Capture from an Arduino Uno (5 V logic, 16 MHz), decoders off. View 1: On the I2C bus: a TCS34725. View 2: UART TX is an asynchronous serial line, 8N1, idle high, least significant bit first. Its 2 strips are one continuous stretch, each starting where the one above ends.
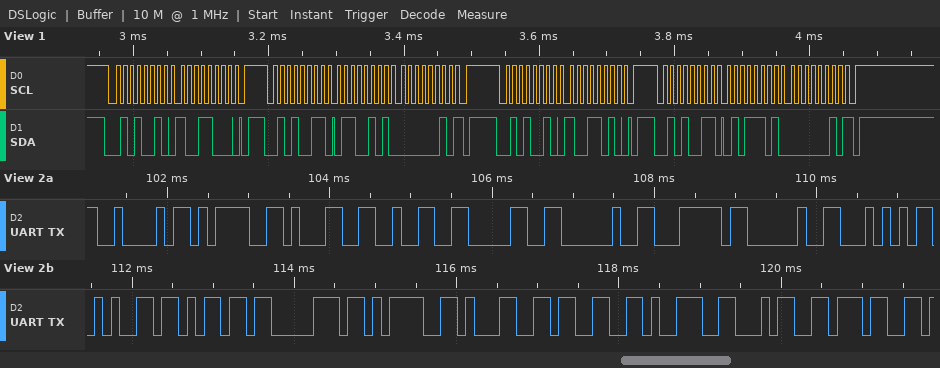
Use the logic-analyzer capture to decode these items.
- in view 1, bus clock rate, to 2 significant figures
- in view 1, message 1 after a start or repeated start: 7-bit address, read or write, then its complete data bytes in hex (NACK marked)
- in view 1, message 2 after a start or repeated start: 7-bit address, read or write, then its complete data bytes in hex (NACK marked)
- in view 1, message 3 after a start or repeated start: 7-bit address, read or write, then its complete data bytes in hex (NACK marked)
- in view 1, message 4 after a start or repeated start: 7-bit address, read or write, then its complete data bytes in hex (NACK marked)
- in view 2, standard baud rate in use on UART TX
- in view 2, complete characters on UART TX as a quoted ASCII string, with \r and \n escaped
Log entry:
100 kHz
0x29 write: 98
0x29 read: 65 02 NACK
0x29 write: 9A
0x29 read: 5D 02 NACK
9600 baud
"B=120 | Temp=13947"
